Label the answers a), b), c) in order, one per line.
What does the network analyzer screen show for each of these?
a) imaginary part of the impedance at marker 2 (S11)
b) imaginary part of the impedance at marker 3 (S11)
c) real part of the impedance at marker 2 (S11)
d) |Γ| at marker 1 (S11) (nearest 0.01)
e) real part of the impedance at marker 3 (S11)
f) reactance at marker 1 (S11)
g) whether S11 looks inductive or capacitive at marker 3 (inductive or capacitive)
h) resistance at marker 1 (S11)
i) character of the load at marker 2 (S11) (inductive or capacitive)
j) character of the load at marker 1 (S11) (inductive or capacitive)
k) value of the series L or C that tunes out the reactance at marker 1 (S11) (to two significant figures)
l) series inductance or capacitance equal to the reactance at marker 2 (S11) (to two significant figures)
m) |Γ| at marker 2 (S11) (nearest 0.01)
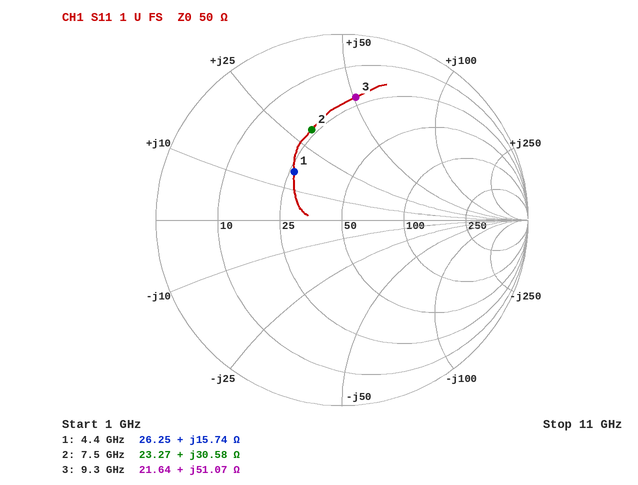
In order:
a) +30.58 Ω
b) +51.07 Ω
c) 23.27 Ω
d) 0.37
e) 21.64 Ω
f) +15.74 Ω
g) inductive
h) 26.25 Ω
i) inductive
j) inductive
k) 2.3 pF
l) 650 pH
m) 0.51
